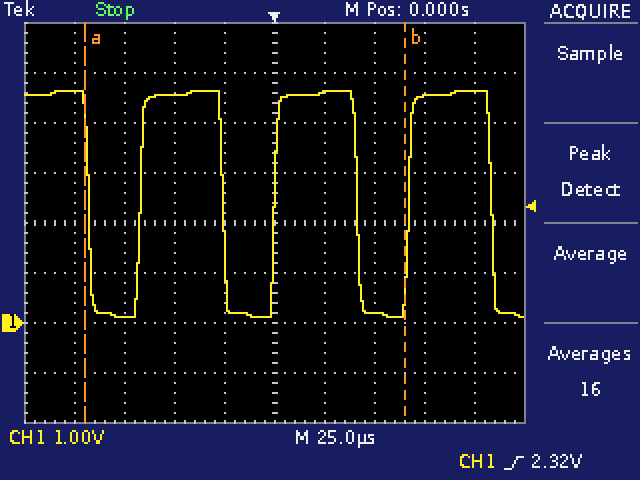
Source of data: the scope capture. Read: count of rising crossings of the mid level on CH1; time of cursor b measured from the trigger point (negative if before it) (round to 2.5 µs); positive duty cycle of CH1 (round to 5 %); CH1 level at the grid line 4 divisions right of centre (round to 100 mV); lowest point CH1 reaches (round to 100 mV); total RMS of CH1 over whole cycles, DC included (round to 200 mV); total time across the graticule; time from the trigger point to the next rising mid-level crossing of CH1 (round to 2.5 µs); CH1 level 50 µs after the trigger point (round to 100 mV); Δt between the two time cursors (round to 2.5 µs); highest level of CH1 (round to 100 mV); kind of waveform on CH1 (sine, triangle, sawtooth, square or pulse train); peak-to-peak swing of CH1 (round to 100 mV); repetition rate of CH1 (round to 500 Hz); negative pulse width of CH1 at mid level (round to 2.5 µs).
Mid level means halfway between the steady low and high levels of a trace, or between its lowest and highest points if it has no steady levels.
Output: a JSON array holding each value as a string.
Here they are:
["3", "+65.0 µs", "60 %", "4.6 V", "100 mV", "3.6 V", "250 µs", "67.5 µs", "200 mV", "160.0 µs", "4.6 V", "pulse train", "4.5 V", "15.0 kHz", "25.0 µs"]
